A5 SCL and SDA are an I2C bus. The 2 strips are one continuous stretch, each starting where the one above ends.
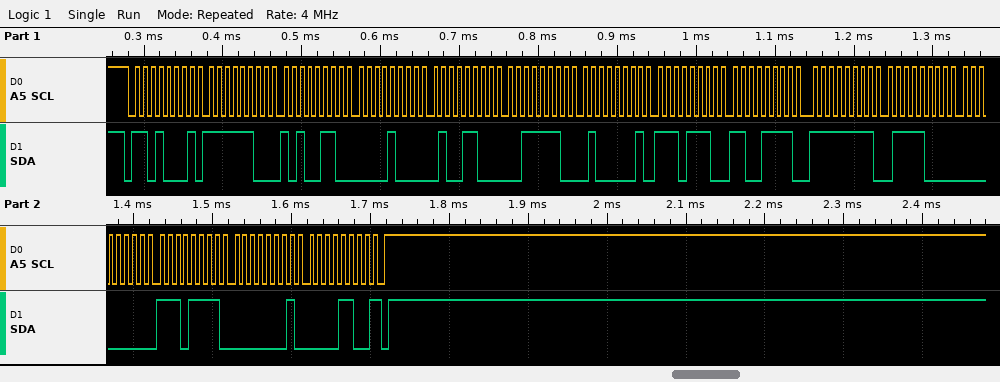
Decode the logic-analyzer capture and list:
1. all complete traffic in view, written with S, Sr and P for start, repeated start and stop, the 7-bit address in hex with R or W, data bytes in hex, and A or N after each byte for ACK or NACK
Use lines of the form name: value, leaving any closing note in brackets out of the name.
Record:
all complete traffic in view, written with S, Sr and P for start, repeated start and stop, the 7-bit address in hex with R or W, data bytes in hex, and A or N after each byte for ACK or NACK: S 68R A FC A A6 A 08 A 4C A 3E A 41 A EE A CF A FF A 78 A 00 A EF A 01 A 0C N P
